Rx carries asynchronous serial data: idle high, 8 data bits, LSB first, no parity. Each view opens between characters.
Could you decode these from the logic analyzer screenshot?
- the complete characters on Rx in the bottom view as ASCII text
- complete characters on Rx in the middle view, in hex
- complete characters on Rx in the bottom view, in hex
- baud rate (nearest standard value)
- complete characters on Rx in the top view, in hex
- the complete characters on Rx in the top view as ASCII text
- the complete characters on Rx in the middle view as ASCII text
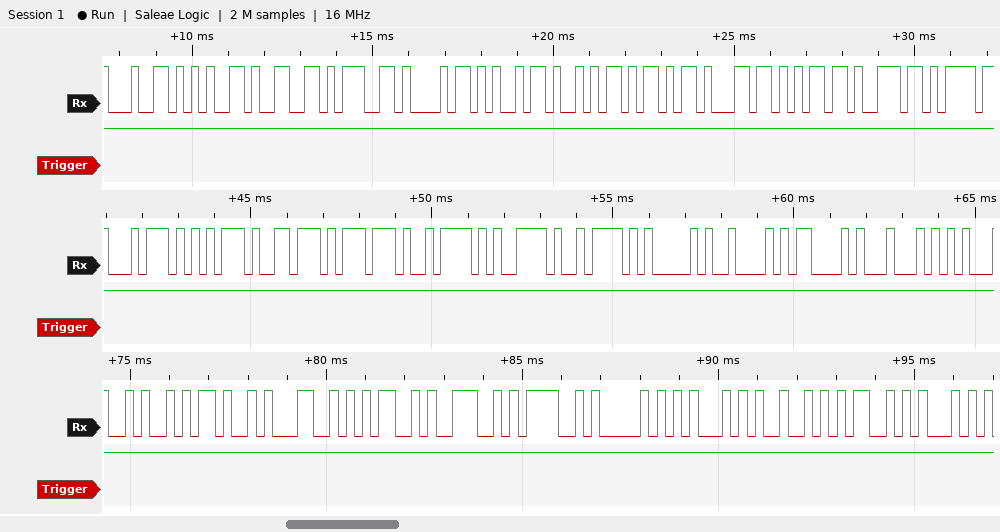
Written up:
"JKLMNOPQRS"
74, 75, 76, 77, 7A, 79, 7A, 41, 42, 43, 44
4A, 4B, 4C, 4D, 4E, 4F, 50, 51, 52, 53
4800 baud
64, 65, 66, 67, 68, 69, 6A, 6B, 6C, 6D, 6E
"defghijklmn"
"tuvwzyzABCD"
